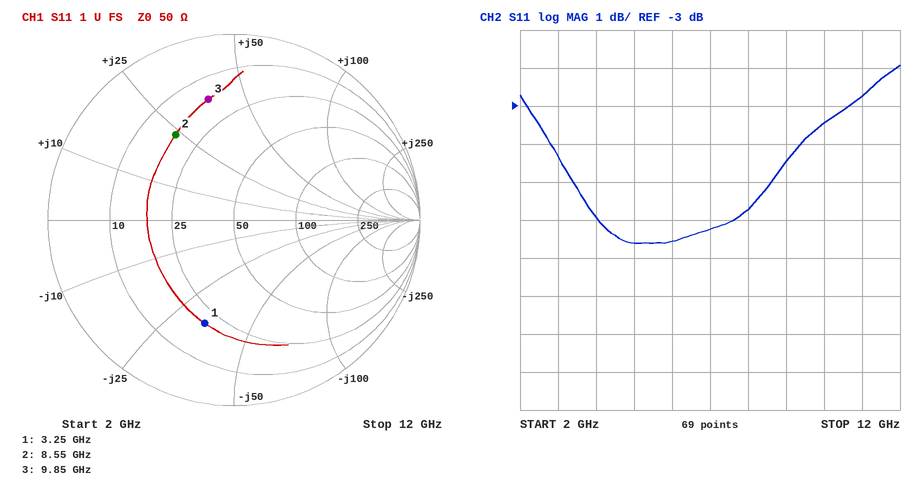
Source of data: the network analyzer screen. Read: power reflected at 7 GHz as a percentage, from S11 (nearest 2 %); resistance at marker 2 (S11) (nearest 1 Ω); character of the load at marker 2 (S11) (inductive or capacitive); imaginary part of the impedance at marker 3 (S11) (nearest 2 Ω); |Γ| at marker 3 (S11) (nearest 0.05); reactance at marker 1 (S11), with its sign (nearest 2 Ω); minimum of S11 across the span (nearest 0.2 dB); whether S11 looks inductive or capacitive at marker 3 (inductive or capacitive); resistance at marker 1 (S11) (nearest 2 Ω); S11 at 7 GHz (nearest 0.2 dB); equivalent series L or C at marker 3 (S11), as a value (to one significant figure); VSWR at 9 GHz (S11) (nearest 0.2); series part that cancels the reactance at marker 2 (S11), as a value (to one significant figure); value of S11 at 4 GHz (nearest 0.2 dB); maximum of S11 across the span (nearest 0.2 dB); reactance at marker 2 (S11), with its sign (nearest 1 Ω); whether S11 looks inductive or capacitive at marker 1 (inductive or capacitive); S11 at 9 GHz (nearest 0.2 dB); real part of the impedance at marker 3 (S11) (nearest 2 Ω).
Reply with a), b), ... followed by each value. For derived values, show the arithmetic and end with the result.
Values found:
a) 10^(-6.2/10) ≈ 24 %
b) 18 Ω
c) inductive
d) +38 Ω
e) 0.65
f) -34 Ω
g) -6.6 dB
h) inductive
i) 20 Ω
j) -6.2 dB
k) L = 38 Ω/(2π × 9.85 GHz) ≈ 614 pH, so 600 pH to one significant figure
l) |Γ| = 10^(-4.4/20) = 0.6026; VSWR = (1 + 0.6026)/(1 − 0.6026) ≈ 4.0
m) C = 1/(2π × 8.55 GHz × 24 Ω) ≈ 776 fF, so 800 fF to one significant figure
n) -6.0 dB
o) -2.0 dB
p) +24 Ω
q) capacitive
r) -4.4 dB
s) 16 Ω
